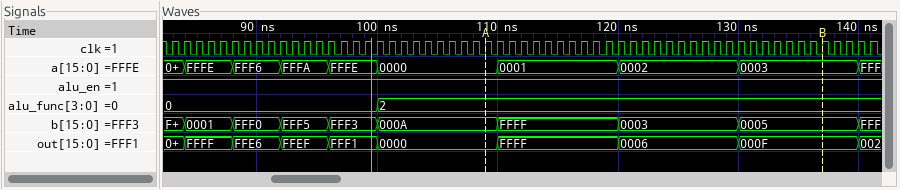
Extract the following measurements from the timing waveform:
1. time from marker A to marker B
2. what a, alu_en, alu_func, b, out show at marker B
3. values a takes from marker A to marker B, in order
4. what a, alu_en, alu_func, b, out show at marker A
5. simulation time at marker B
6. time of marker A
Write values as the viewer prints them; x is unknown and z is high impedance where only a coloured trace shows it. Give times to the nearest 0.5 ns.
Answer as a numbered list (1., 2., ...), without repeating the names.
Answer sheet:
1. 28 ns
2. a=0003, alu_en=1, alu_func=2, b=0005, out=000F
3. 0000, 0001, 0002, 0003
4. a=0000, alu_en=1, alu_func=2, b=000A, out=0000
5. 137 ns
6. 109 ns
